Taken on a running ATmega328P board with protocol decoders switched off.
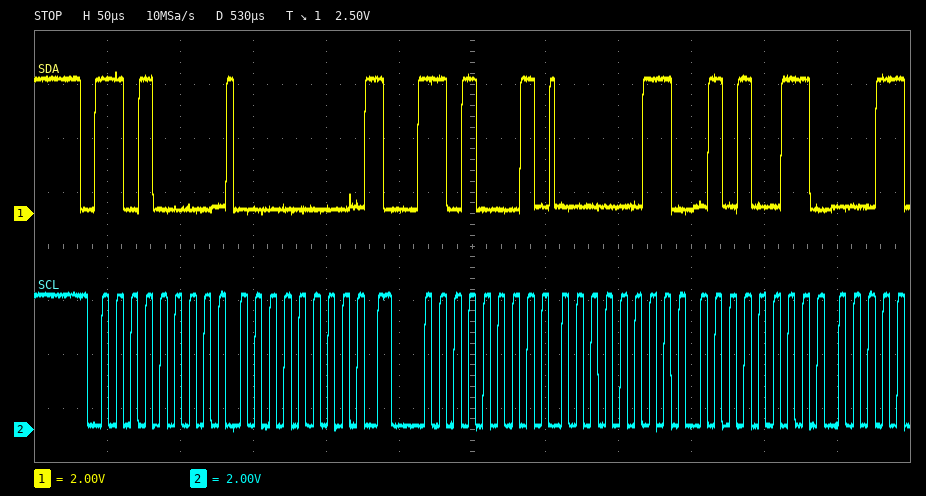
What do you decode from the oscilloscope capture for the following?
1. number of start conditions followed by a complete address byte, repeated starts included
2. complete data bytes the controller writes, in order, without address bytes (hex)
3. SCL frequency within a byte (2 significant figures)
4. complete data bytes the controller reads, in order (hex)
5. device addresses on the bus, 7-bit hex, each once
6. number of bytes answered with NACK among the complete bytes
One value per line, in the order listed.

2
00
100 kHz
03 53
0x68
0
